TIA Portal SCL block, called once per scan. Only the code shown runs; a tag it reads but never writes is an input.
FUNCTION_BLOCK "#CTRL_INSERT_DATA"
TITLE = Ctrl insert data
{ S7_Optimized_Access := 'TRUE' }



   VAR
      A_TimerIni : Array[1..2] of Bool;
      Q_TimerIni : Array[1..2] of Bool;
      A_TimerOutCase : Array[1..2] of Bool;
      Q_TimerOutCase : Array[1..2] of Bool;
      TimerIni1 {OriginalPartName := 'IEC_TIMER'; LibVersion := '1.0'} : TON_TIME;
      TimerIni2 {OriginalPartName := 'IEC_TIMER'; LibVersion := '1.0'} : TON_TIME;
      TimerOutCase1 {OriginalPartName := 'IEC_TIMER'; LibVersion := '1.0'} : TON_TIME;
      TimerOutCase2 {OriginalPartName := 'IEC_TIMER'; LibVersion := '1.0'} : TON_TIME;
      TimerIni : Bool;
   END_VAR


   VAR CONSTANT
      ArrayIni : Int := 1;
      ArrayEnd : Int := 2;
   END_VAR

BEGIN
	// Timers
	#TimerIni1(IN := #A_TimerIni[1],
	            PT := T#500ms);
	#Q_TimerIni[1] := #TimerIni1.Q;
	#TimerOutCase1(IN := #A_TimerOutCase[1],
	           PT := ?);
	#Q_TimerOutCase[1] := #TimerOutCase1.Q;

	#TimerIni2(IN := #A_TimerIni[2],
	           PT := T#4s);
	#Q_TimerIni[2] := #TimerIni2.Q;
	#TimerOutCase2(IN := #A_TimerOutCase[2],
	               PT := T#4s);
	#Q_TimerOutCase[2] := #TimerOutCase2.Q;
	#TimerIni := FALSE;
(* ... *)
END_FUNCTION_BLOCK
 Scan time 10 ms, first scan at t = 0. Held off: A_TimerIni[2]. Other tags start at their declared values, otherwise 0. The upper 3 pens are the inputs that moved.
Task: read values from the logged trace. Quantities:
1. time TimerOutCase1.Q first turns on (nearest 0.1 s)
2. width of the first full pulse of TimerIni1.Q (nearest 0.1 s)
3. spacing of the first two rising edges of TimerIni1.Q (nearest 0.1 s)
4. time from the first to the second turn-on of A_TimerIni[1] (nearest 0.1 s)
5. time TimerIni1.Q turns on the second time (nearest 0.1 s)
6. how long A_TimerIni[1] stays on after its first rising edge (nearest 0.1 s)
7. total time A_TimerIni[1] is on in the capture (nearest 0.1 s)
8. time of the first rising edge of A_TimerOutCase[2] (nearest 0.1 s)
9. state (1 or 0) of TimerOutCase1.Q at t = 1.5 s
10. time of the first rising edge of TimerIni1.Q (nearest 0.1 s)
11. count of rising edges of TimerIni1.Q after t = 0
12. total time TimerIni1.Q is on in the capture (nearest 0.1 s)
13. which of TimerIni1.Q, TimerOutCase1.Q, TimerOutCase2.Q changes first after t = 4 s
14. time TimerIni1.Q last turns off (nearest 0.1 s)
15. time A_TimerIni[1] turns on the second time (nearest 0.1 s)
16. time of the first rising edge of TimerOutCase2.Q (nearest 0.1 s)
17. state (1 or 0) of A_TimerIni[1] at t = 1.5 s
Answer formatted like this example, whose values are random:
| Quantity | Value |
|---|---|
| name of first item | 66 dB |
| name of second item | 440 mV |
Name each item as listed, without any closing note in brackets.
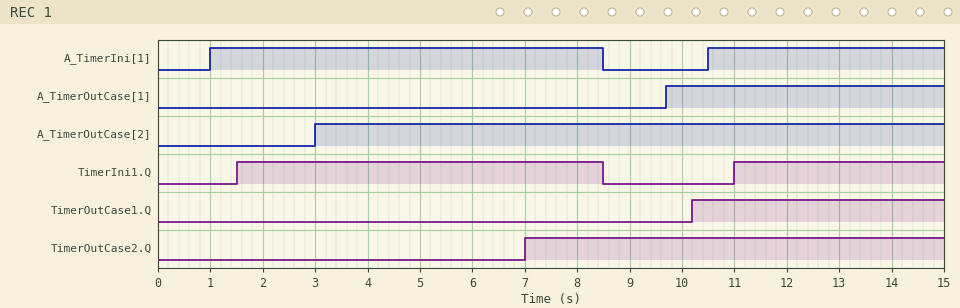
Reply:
| Quantity | Value |
|---|---|
| time TimerOutCase1.Q first turns on | 10.2 s |
| width of the first full pulse of TimerIni1.Q | 7.0 s |
| spacing of the first two rising edges of TimerIni1.Q | 9.5 s |
| time from the first to the second turn-on of A_TimerIni[1] | 9.5 s |
| time TimerIni1.Q turns on the second time | 11.0 s |
| how long A_TimerIni[1] stays on after its first rising edge | 7.5 s |
| total time A_TimerIni[1] is on in the capture | 12.0 s |
| time of the first rising edge of A_TimerOutCase[2] | 3.0 s |
| state (1 or 0) of TimerOutCase1.Q at t = 1.5 s | 0 |
| time of the first rising edge of TimerIni1.Q | 1.5 s |
| count of rising edges of TimerIni1.Q after t = 0 | 2 |
| total time TimerIni1.Q is on in the capture | 11.0 s |
| which of TimerIni1.Q, TimerOutCase1.Q, TimerOutCase2.Q changes first after t = 4 s | TimerOutCase2.Q |
| time TimerIni1.Q last turns off | 8.5 s |
| time A_TimerIni[1] turns on the second time | 10.5 s |
| time of the first rising edge of TimerOutCase2.Q | 7.0 s |
| state (1 or 0) of A_TimerIni[1] at t = 1.5 s | 1 |
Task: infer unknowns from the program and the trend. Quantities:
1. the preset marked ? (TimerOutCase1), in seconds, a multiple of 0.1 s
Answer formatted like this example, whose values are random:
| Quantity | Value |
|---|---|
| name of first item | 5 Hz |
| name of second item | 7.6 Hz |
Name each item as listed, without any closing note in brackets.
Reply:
| Quantity | Value |
|---|---|
| the preset marked ? (TimerOutCase1), in seconds, a multiple of 0.1 s | 0.5 s |
